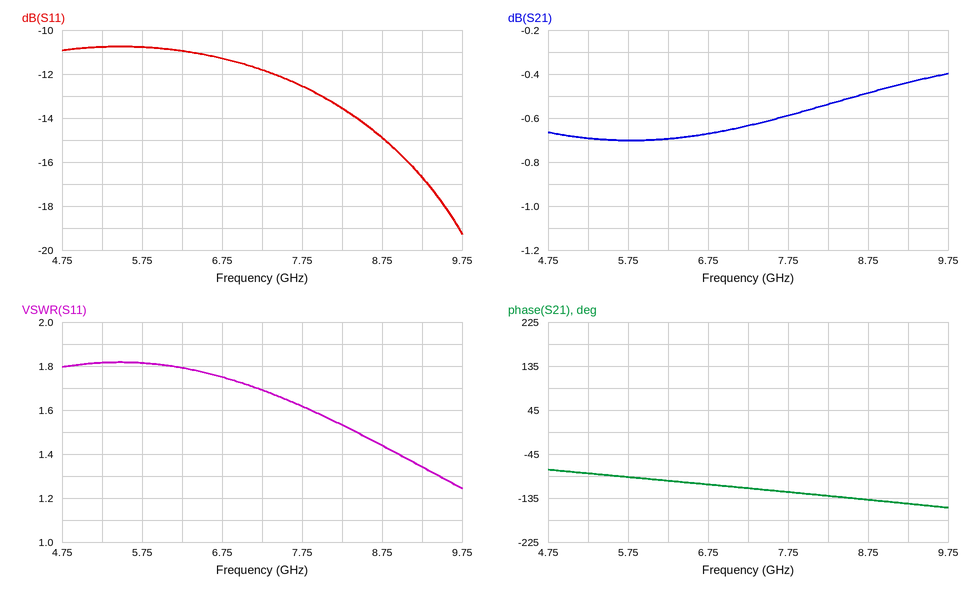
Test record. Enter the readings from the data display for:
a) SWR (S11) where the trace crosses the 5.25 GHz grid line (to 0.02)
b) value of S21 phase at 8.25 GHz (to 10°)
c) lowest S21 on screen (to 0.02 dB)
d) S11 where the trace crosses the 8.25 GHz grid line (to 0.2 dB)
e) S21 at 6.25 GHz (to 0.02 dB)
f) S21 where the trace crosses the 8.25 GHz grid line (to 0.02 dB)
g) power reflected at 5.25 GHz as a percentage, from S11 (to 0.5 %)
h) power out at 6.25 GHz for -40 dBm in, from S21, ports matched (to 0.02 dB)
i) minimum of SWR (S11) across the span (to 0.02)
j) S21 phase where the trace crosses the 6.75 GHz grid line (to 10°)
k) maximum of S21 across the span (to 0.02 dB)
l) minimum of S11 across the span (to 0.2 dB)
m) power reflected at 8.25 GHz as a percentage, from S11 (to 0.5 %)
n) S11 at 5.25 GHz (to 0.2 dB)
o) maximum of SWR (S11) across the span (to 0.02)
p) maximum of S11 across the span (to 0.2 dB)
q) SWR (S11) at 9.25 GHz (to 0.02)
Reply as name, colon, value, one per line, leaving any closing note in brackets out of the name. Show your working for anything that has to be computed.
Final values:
SWR (S11) where the trace crosses the 5.25 GHz grid line: 1.82
value of S21 phase at 8.25 GHz: -130°
lowest S21 on screen: -0.70 dB
S11 where the trace crosses the 8.25 GHz grid line: -13.6 dB
S21 at 6.25 GHz: -0.70 dB
S21 where the trace crosses the 8.25 GHz grid line: -0.54 dB
power reflected at 5.25 GHz as a percentage, from S11: 10^(-10.8/10) ≈ 8.32 %, so 8.5 % to the nearest 0.5 %
power out at 6.25 GHz for -40 dBm in, from S21, ports matched: -40 dBm + (-0.70 dB) = -40.70 dBm
minimum of SWR (S11) across the span: 1.24
S21 phase where the trace crosses the 6.75 GHz grid line: -110°
maximum of S21 across the span: -0.40 dB
minimum of S11 across the span: -19.2 dB
power reflected at 8.25 GHz as a percentage, from S11: 10^(-13.6/10) ≈ 4.37 %, so 4.5 % to the nearest 0.5 %
S11 at 5.25 GHz: -10.8 dB
maximum of SWR (S11) across the span: 1.82
maximum of S11 across the span: -10.8 dB
SWR (S11) at 9.25 GHz: 1.34
